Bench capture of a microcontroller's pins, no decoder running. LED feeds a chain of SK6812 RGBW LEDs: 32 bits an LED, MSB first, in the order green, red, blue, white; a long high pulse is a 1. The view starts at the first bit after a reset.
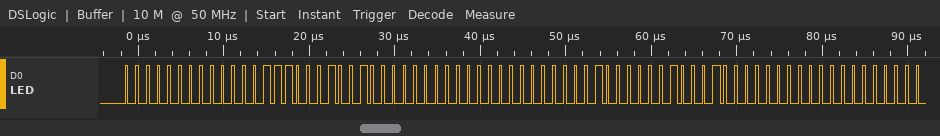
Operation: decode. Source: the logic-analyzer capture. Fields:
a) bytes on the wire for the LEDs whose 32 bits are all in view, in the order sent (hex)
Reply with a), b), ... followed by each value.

a) 00 07 12 00 00 08 11 00
